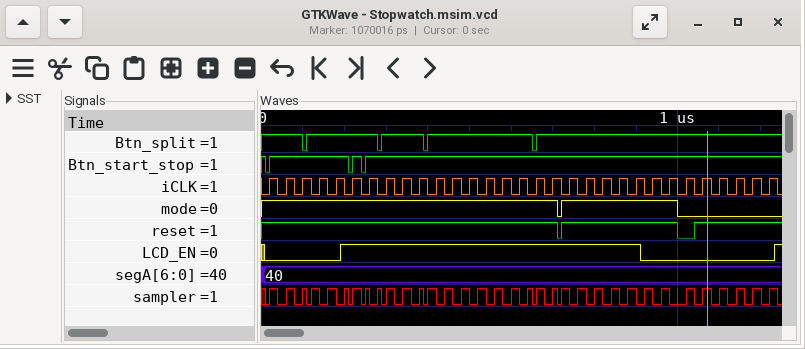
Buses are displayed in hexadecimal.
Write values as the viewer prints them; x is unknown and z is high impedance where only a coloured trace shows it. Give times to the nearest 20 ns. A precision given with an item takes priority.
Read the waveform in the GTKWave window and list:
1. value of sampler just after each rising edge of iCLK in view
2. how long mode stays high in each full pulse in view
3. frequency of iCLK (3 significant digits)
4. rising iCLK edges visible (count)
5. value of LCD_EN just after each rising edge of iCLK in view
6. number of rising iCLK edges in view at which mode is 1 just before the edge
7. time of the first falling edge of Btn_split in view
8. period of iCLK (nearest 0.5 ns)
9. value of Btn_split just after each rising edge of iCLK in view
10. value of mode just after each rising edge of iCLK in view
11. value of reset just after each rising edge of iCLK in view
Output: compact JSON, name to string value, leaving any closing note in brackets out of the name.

{"value of sampler just after each rising edge of iCLK in view": "1 1 1 0 0 1 0 1 1 1 0 0 0 0 0 0 1 1 0 0 0 0 0 0 0 1 1 1 1 1 1", "how long mode stays high in each full pulse in view": "280 ns", "frequency of iCLK": "25.0 MHz", "rising iCLK edges visible": "31", "value of LCD_EN just after each rising edge of iCLK in view": "0 0 0 0 0 1 1 1 1 1 1 1 1 1 1 1 1 1 1 1 1 1 1 0 0 0 0 0 0 0 0", "number of rising iCLK edges in view at which mode is 1 just before the edge": "25", "time of the first falling edge of Btn_split in view": "100 ns", "period of iCLK": "40 ns", "value of Btn_split just after each rising edge of iCLK in view": "1 1 0 1 1 1 1 1 1 1 1 1 1 1 1 1 1 1 1 1 1 1 1 1 1 1 1 1 1 1 1", "value of mode just after each rising edge of iCLK in view": "1 1 1 1 1 1 1 1 1 1 1 1 1 1 1 1 1 1 1 1 1 1 1 1 1 0 0 0 0 0 0", "value of reset just after each rising edge of iCLK in view": "1 1 1 1 1 1 1 1 1 1 1 1 1 1 1 1 1 1 1 1 1 1 1 1 1 0 1 1 1 1 1"}
